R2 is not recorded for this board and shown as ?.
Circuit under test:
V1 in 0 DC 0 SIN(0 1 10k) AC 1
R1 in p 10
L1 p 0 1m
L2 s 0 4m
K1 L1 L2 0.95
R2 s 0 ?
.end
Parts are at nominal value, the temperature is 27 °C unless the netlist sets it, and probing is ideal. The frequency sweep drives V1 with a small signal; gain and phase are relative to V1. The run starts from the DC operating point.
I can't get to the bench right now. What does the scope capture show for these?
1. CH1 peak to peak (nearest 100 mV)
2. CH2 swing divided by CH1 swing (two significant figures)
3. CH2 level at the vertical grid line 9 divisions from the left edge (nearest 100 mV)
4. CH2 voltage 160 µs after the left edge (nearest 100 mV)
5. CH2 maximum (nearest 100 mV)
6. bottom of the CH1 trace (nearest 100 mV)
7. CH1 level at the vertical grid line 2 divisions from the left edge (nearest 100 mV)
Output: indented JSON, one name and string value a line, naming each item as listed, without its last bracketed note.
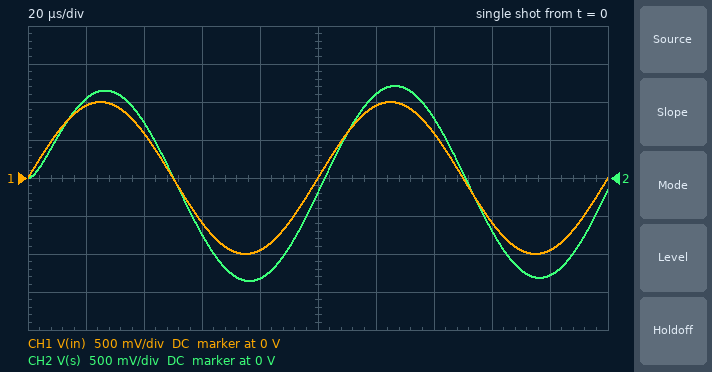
{
  "CH1 peak to peak": "2.0 V",
  "CH2 swing divided by CH1 swing": "1.3",
  "CH2 level at the vertical grid line 9 divisions from the left edge": "-1.3 V",
  "CH2 voltage 160 µs after the left edge": "-700 mV",
  "CH2 maximum": "1.2 V",
  "bottom of the CH1 trace": "-1.0 V",
  "CH1 level at the vertical grid line 2 divisions from the left edge": "600 mV"
}
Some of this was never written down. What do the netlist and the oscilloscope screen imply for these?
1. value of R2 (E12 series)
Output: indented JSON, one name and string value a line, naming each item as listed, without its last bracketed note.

{
  "value of R2": "82 Ω"
}
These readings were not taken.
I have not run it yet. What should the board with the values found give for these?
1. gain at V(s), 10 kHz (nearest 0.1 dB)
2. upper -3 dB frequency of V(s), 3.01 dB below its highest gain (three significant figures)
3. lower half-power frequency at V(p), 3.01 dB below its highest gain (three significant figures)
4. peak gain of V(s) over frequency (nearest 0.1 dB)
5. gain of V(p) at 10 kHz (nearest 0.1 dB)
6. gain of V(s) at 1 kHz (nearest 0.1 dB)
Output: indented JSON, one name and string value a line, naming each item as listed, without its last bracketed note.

{
  "gain at V(s), 10 kHz": "2.1 dB",
  "upper -3 dB frequency of V(s), 3.01 dB below its highest gain": "50.8 kHz",
  "lower half-power frequency at V(p), 3.01 dB below its highest gain": "12.3 kHz",
  "peak gain of V(s) over frequency": "2.1 dB",
  "gain of V(p) at 10 kHz": "-3.1 dB",
  "gain of V(s) at 1 kHz": "-1.1 dB"
}
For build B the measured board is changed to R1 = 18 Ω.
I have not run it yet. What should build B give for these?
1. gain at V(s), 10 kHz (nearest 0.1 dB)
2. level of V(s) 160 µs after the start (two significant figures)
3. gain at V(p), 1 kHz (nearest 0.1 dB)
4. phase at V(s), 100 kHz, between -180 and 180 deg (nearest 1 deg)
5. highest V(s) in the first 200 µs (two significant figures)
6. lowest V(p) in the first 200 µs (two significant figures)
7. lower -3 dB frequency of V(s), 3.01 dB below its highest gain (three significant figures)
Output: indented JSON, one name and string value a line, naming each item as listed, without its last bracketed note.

{
  "gain at V(s), 10 kHz": "0.1 dB",
  "level of V(s) 160 µs after the start": "-620 mV",
  "gain at V(p), 1 kHz": "-10.6 dB",
  "phase at V(s), 100 kHz, between -180 and 180 deg": "-58 deg",
  "highest V(s) in the first 200 µs": "960 mV",
  "lowest V(p) in the first 200 µs": "-600 mV",
  "lower -3 dB frequency of V(s), 3.01 dB below its highest gain": "1.49 kHz"
}
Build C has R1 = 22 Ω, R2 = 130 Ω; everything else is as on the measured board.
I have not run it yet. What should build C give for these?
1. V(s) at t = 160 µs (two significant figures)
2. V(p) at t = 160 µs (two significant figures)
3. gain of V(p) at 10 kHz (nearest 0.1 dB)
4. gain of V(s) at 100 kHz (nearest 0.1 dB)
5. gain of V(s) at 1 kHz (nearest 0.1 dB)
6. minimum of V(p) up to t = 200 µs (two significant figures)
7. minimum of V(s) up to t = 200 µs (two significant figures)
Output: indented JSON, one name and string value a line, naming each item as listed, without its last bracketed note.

{
  "V(s) at t = 160 µs": "-780 mV",
  "V(p) at t = 160 µs": "-490 mV",
  "gain of V(p) at 10 kHz": "-4.4 dB",
  "gain of V(s) at 100 kHz": "-2.4 dB",
  "gain of V(s) at 1 kHz": "-6.2 dB",
  "minimum of V(p) up to t = 200 µs": "-650 mV",
  "minimum of V(s) up to t = 200 µs": "-1.2 V"
}
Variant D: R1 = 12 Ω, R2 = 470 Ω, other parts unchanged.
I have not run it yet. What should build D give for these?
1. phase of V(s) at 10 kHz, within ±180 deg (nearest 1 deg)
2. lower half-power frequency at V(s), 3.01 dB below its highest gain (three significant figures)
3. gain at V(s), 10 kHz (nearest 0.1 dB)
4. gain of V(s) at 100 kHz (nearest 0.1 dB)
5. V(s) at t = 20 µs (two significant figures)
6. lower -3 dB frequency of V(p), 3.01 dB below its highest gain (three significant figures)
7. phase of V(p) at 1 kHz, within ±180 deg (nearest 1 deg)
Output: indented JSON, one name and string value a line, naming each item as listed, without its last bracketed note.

{
  "phase of V(s) at 10 kHz, within ±180 deg": "7 deg",
  "lower half-power frequency at V(s), 3.01 dB below its highest gain": "1.72 kHz",
  "gain at V(s), 10 kHz": "4.7 dB",
  "gain of V(s) at 100 kHz": "3.9 dB",
  "V(s) at t = 20 µs": "1.4 V",
  "lower -3 dB frequency of V(p), 3.01 dB below its highest gain": "2.13 kHz",
  "phase of V(p) at 1 kHz, within ±180 deg": "60 deg"
}
